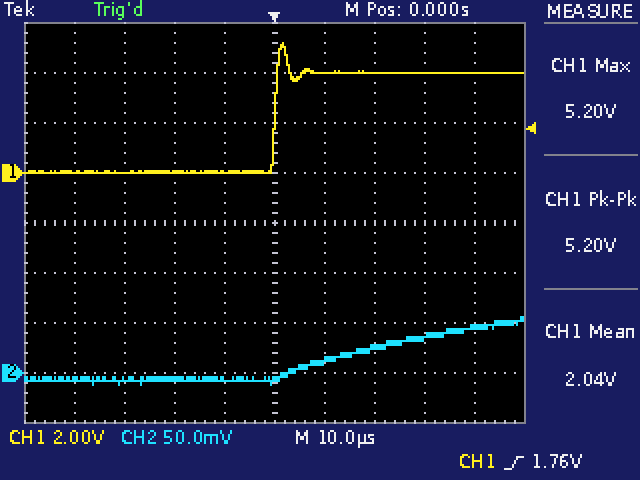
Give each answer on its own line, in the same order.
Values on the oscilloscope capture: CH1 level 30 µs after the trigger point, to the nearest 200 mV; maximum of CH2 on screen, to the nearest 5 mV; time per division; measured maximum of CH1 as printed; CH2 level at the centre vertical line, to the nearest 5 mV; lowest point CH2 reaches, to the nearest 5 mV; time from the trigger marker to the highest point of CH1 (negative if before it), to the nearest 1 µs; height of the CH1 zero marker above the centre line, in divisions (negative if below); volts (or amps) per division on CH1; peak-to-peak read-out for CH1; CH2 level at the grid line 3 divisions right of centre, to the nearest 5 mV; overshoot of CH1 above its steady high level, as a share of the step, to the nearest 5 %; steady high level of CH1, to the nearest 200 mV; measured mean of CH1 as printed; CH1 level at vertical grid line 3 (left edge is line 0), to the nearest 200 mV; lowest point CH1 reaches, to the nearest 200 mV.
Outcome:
4.0 V
55 mV
10 µs
5.20 V
-10 mV
-10 mV
+2 µs
+1.0 div
2 V
5.20 V
35 mV
30 %
4.0 V
2.04 V
0.0 V
0.0 V
